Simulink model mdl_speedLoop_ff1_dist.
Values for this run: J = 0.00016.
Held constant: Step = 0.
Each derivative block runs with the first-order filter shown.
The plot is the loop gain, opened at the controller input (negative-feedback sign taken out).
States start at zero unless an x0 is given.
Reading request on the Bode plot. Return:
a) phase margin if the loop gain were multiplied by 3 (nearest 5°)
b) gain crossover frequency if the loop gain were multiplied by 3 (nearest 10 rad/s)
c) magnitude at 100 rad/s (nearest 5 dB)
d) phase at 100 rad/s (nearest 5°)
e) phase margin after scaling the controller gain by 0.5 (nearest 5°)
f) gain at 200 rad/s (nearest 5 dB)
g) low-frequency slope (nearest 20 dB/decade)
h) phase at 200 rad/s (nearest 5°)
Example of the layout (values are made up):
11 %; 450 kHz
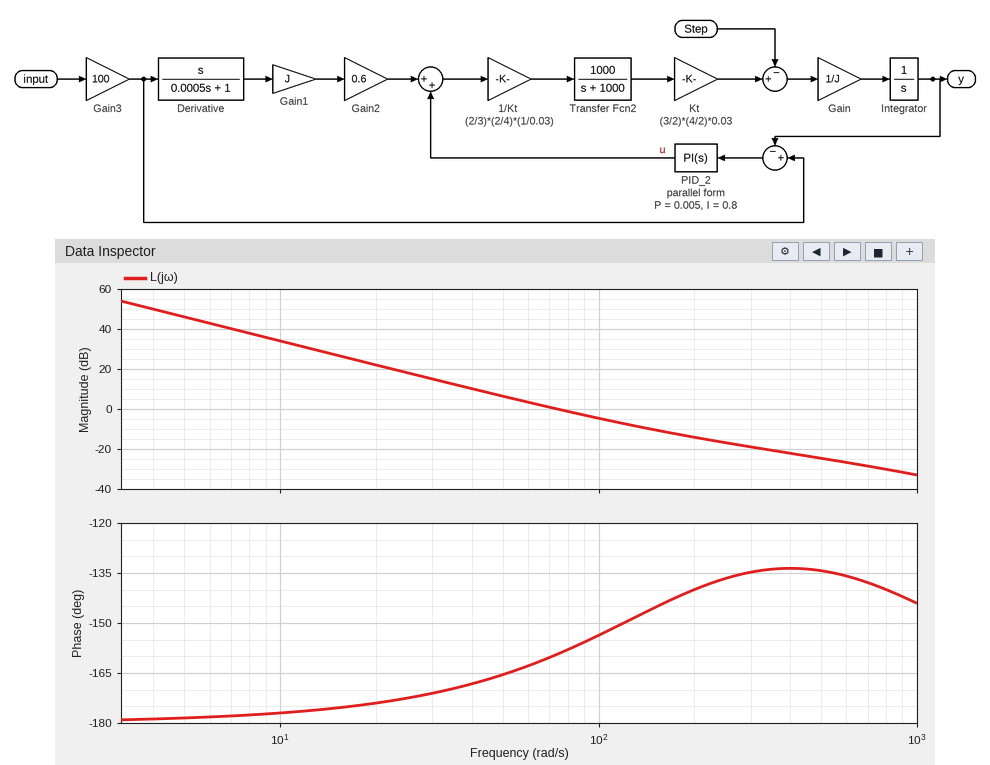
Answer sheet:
35°; 140 rad/s; -5 dB; -155°; 15°; -15 dB; -40 dB/decade; -140°
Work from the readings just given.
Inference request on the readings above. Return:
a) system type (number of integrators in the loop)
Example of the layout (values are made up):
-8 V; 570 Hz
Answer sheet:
2
